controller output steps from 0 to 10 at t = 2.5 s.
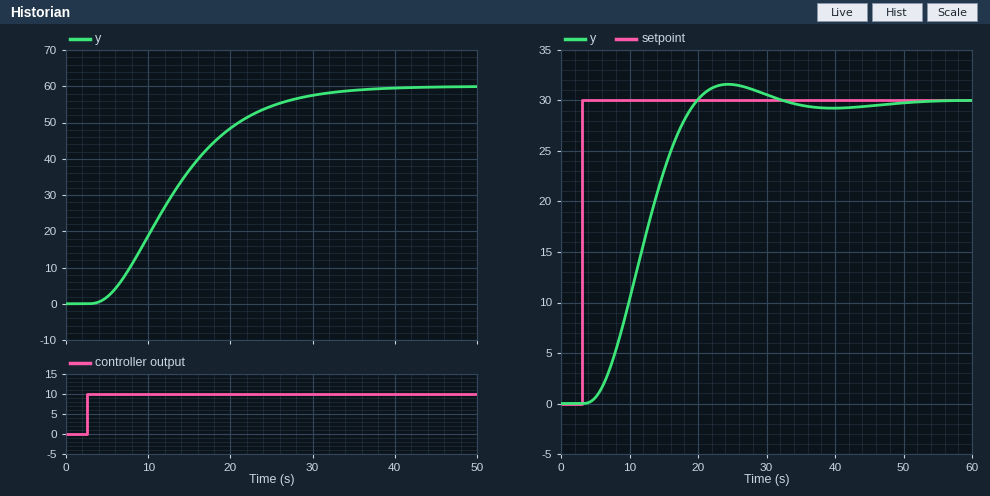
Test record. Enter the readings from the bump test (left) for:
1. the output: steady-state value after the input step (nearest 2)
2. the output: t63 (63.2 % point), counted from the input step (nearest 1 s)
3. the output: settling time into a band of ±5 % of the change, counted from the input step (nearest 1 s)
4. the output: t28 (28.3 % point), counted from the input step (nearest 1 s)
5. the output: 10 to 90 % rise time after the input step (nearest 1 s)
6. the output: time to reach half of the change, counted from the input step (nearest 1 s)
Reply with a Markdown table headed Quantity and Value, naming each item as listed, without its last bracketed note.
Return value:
| Quantity | Value |
|---|---|
| the output: steady-state value after the input step | 60 |
| the output: t63 (63.2 % point), counted from the input step | 13 s |
| the output: settling time into a band of ±5 % of the change, counted from the input step | 26 s |
| the output: t28 (28.3 % point), counted from the input step | 7 s |
| the output: 10 to 90 % rise time after the input step | 18 s |
| the output: time to reach half of the change, counted from the input step | 10 s |
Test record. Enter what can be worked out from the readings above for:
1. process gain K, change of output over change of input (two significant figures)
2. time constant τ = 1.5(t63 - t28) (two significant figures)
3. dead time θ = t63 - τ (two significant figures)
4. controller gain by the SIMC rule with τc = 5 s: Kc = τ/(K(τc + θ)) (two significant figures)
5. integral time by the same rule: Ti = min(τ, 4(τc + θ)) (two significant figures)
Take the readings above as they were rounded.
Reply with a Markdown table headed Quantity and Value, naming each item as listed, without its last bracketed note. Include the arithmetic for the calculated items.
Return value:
| Quantity | Value |
|---|---|
| process gain K, change of output over change of input | (60 - 0) / 10 = 6.0 |
| time constant τ = 1.5(t63 - t28) | 1.5 × (13 - 7) = 9.0 s |
| dead time θ = t63 - τ | 13 - 9 = 4.0 s |
| controller gain by the SIMC rule with τc = 5 s: Kc = τ/(K(τc + θ)) | 9 / (6 × (5 + 4)) = 0.17 |
| integral time by the same rule: Ti = min(τ, 4(τc + θ)) | min(9, 4 × (5 + 4)) = 9.0 s |
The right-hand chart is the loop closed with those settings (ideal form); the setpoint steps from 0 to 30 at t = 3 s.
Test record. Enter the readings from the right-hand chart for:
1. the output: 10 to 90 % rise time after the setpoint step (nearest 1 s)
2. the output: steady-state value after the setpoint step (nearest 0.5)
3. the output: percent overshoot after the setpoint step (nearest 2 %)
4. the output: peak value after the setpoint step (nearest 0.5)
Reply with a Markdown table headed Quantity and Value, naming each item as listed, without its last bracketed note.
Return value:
| Quantity | Value |
|---|---|
| the output: 10 to 90 % rise time after the setpoint step | 10 s |
| the output: steady-state value after the setpoint step | 30.0 |
| the output: percent overshoot after the setpoint step | 6 % |
| the output: peak value after the setpoint step | 31.5 |
